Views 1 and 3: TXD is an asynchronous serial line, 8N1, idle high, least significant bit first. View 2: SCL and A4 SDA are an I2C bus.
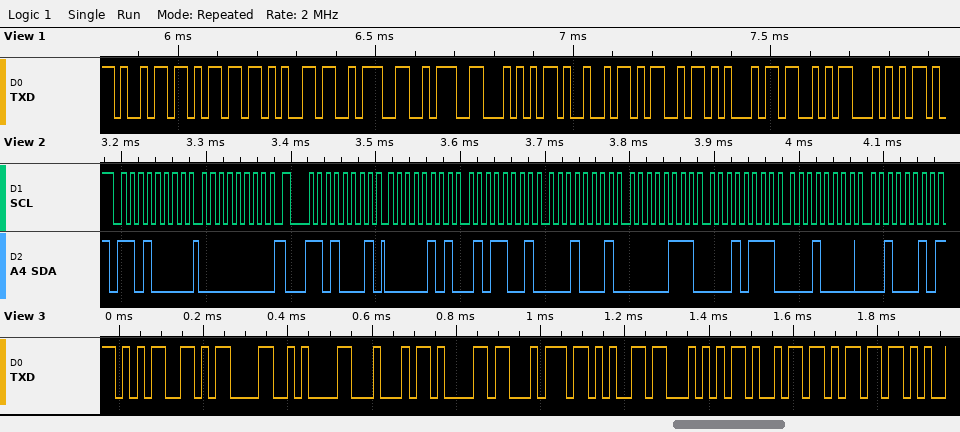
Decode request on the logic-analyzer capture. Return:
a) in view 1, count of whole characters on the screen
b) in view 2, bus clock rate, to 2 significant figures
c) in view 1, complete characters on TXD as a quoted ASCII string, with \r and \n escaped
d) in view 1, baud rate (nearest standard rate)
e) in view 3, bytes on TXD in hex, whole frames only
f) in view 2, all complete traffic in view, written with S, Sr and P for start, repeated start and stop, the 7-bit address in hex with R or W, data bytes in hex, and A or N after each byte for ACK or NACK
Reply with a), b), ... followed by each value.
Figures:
a) 11
b) 100 kHz
c) "ime::TIMEST"
d) 57600 baud
e) 0x35 0x0D 0x0A 0x44 0x61 0x74 0x65 0x54 0x69 0x6D
f) S 68W A 00 A Sr 68R A 05 A 59 A 11 A 07 A 17 A 10 A 22 N
